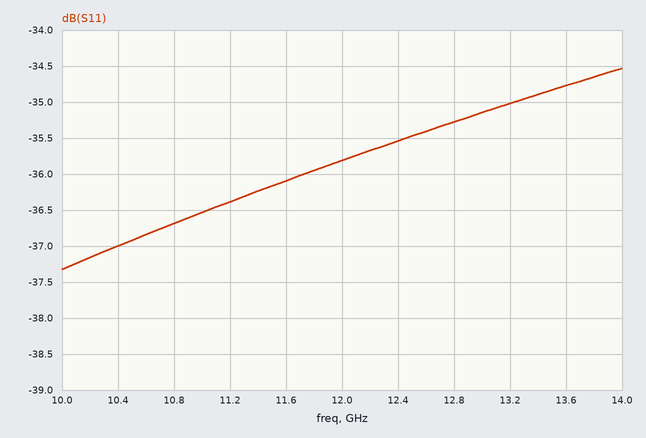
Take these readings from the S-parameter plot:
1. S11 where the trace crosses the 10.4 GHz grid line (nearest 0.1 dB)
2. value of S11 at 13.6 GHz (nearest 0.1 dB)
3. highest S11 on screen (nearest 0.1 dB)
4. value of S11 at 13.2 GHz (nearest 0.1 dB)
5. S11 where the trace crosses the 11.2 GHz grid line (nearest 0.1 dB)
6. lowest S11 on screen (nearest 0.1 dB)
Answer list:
-37.0 dB
-34.8 dB
-34.5 dB
-35.0 dB
-36.4 dB
-37.3 dB
